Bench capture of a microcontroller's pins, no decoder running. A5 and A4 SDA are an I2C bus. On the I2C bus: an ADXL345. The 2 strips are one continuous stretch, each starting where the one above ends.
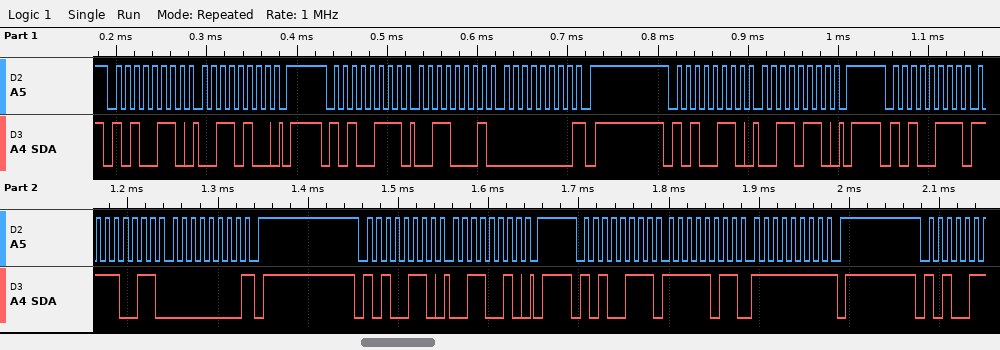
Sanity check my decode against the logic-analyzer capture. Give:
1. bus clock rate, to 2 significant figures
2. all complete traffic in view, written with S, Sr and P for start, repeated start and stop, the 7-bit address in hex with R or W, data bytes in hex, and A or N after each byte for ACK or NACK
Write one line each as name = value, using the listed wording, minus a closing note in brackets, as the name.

bus clock rate, to 2 significant figures = 100 kHz
all complete traffic in view, written with S, Sr and P for start, repeated start and stop, the 7-bit address in hex with R or W, data bytes in hex, and A or N after each byte for ACK or NACK = S 53W A 34 A P S 53R A 31 A 00 N P S 53W A 36 A P S 53R A F3 A 00 N P S 53W A 32 A P S 53R A FB A FF N P
